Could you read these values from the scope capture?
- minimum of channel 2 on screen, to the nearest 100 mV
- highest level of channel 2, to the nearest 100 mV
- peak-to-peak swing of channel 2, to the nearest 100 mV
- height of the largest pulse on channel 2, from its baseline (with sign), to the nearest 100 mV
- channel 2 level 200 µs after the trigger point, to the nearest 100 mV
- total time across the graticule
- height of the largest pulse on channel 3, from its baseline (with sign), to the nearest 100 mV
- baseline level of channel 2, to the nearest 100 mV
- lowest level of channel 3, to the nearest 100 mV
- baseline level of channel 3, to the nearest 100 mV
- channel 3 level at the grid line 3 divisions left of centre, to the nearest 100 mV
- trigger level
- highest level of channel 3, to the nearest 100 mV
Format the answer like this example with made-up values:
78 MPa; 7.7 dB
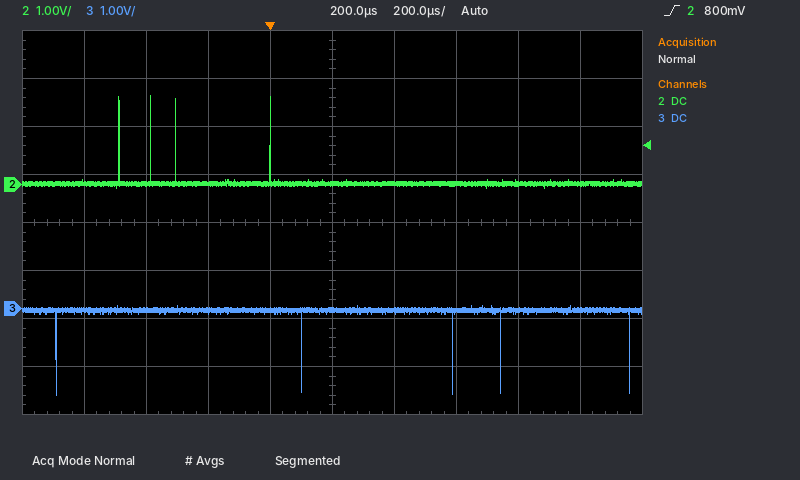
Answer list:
-100 mV; 1.8 V; 1.9 V; +1.8 V; 0.0 V; 2 ms; -1.8 V; 0.0 V; -1.8 V; 0.0 V; 0.0 V; 800 mV; 100 mV
